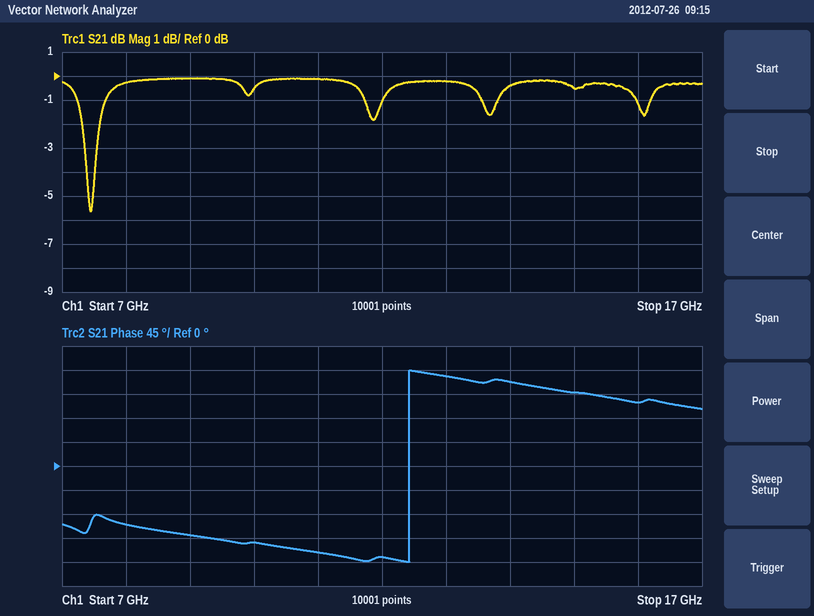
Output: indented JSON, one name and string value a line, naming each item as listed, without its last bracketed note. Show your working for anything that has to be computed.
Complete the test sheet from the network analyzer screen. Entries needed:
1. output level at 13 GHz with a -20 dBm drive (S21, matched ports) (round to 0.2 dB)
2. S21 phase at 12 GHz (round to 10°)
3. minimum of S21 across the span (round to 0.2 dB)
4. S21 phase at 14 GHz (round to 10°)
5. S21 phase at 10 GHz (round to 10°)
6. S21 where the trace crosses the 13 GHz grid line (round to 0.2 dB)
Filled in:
{
  "output level at 13 GHz with a -20 dBm drive (S21, matched ports)": "-20 dBm + (-0.2 dB) = -20.2 dBm",
  "S21 phase at 12 GHz": "-170°",
  "minimum of S21 across the span": "-5.6 dB",
  "S21 phase at 14 GHz": "160°",
  "S21 phase at 10 GHz": "-140°",
  "S21 where the trace crosses the 13 GHz grid line": "-0.2 dB"
}
